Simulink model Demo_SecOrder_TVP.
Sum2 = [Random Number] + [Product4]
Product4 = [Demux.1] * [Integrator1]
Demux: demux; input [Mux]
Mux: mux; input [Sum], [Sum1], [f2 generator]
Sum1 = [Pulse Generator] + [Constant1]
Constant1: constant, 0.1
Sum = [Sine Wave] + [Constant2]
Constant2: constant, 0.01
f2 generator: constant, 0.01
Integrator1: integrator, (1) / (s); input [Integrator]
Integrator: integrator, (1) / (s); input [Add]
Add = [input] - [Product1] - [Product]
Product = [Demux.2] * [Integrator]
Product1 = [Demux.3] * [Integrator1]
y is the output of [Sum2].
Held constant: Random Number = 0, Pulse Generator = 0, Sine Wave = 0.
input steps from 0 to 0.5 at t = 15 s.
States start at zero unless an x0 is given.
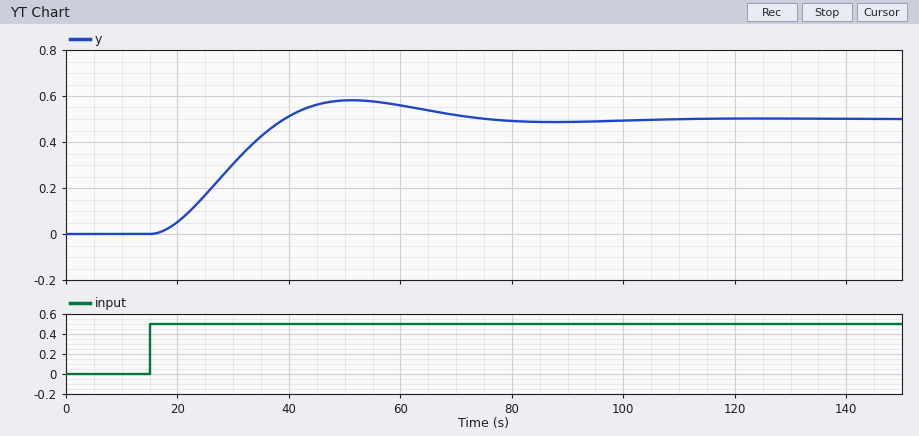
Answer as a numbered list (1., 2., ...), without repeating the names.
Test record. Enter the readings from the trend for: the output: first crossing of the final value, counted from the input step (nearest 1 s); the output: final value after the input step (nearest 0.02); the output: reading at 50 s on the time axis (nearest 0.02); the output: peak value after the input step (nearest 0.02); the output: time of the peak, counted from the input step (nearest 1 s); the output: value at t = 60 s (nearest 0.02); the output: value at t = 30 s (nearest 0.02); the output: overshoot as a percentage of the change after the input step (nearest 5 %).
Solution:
1. 24 s
2. 0.50
3. 0.58
4. 0.58
5. 36 s
6. 0.56
7. 0.30
8. 15 %
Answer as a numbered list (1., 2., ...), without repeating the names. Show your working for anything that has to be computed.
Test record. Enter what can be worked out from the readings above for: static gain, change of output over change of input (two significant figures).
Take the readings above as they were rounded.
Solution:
1. (0.5 - 0) / (0.5 - 0) = 1.0
